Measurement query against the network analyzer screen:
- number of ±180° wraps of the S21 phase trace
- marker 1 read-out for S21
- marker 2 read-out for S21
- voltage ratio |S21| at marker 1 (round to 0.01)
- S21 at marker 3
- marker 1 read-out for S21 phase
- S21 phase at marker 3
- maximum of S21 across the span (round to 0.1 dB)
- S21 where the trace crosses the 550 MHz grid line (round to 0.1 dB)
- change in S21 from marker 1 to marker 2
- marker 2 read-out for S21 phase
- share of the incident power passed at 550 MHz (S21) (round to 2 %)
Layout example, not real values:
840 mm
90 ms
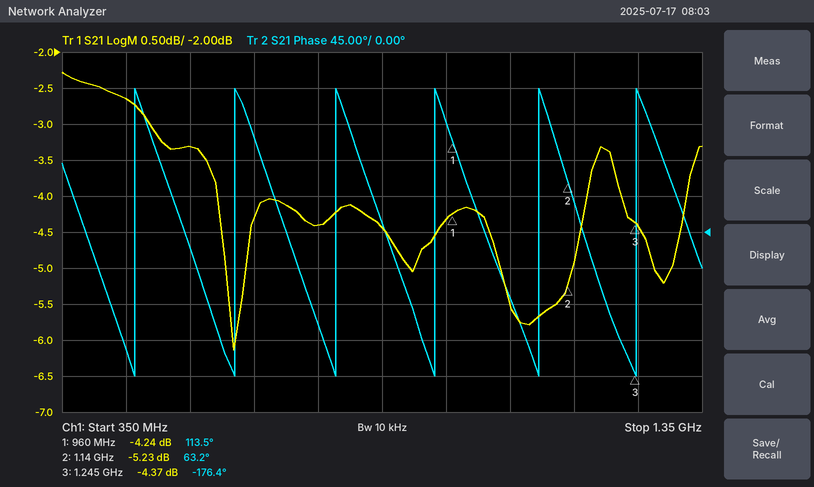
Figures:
6
-4.24 dB
-5.23 dB
0.61
-4.37 dB
113.5°
-176.4°
-2.3 dB
-3.3 dB
-0.99 dB
63.2°
46 %
